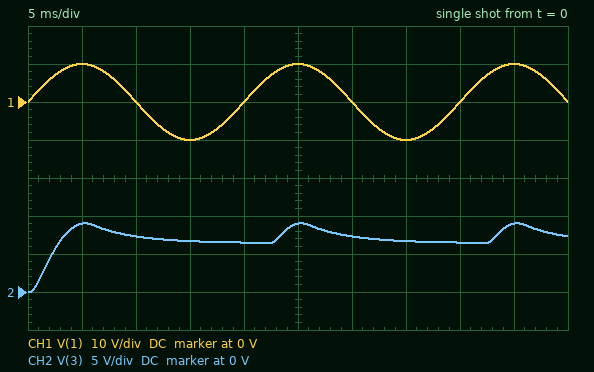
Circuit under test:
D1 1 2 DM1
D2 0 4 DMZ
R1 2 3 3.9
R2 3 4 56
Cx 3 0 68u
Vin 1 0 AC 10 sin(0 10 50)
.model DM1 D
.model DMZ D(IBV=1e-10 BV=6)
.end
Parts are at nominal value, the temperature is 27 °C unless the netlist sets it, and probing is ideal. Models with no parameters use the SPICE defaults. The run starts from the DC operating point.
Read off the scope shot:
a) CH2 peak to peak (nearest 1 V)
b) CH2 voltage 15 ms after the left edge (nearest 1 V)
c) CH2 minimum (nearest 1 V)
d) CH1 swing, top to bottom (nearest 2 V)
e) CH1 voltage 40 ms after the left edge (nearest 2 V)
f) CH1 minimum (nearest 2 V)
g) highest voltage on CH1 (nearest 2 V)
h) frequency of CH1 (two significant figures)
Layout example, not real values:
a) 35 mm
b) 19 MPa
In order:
a) 9 V
b) 7 V
c) 0 V
d) 20 V
e) 0 V
f) -10 V
g) 10 V
h) 50 Hz
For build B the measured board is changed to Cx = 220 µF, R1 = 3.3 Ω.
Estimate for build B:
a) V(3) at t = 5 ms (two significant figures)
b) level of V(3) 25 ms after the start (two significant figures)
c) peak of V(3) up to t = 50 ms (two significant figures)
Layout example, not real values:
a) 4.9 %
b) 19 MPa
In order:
a) 8.6 V
b) 8.7 V
c) 8.9 V
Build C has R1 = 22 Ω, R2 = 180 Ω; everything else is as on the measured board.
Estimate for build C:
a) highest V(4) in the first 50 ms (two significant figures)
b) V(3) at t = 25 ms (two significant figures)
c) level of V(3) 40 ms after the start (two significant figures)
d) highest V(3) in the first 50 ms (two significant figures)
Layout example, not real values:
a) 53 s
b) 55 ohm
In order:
a) 6.5 V
b) 8.2 V
c) 7.1 V
d) 8.5 V
